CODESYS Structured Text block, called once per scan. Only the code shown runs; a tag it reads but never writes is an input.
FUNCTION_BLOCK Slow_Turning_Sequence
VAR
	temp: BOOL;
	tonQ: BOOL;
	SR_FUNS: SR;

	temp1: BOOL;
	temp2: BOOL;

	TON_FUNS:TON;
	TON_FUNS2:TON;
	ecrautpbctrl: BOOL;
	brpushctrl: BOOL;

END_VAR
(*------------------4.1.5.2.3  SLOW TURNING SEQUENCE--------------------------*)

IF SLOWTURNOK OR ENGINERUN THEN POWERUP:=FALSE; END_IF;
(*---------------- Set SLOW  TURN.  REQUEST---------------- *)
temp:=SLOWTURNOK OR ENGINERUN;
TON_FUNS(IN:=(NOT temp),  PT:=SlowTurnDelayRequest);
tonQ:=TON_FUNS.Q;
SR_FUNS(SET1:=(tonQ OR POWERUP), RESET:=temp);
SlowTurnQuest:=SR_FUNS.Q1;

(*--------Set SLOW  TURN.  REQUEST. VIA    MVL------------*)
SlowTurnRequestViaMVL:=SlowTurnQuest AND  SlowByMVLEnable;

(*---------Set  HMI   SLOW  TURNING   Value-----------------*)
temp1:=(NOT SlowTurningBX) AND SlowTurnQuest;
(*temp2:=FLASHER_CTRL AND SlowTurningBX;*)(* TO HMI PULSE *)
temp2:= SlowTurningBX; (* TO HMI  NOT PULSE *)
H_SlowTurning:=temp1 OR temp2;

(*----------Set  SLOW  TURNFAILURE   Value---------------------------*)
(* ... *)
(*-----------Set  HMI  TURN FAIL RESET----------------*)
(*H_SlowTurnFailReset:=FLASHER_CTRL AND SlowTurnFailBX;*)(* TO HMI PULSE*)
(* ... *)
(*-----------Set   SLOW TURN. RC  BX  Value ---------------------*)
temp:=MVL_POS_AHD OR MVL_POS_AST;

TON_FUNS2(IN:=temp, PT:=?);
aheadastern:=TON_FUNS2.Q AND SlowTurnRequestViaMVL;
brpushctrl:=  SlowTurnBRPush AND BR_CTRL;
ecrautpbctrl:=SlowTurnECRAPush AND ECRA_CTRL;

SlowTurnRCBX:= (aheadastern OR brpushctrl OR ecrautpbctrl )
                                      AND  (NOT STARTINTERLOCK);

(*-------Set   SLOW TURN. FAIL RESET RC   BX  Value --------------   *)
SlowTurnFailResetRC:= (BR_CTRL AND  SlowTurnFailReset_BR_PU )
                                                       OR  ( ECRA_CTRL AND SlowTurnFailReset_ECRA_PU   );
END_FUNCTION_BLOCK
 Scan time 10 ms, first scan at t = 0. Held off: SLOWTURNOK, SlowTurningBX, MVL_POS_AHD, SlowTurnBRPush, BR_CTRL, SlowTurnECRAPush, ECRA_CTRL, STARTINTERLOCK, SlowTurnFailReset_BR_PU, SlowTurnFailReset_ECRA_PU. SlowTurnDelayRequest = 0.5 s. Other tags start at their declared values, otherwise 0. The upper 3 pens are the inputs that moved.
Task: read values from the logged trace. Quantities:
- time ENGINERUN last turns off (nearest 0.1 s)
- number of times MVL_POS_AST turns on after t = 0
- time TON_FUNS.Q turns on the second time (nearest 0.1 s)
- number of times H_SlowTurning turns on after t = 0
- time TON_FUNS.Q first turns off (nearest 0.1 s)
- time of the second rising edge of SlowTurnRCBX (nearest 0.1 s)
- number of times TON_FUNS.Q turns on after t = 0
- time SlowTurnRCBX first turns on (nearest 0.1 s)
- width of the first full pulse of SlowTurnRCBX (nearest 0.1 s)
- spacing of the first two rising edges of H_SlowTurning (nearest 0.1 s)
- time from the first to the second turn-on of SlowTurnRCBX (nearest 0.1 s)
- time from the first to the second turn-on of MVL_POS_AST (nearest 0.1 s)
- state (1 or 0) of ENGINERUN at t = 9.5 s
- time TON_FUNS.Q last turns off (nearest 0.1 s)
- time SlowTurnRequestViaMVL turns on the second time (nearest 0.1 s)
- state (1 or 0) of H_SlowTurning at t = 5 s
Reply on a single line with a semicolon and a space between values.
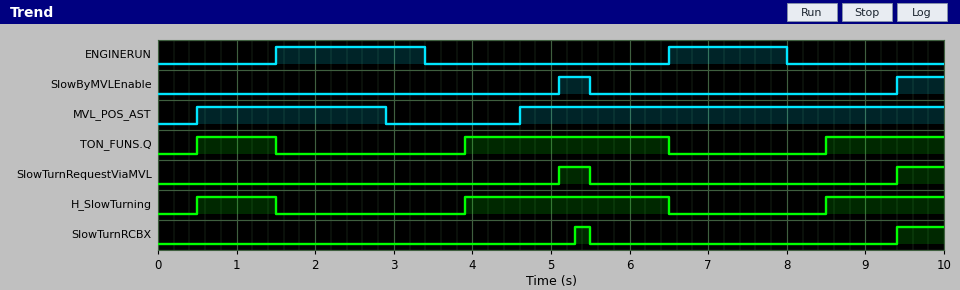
8.0 s; 2; 3.9 s; 3; 1.5 s; 9.4 s; 3; 5.3 s; 0.2 s; 3.4 s; 4.1 s; 4.1 s; 0; 6.5 s; 9.4 s; 1
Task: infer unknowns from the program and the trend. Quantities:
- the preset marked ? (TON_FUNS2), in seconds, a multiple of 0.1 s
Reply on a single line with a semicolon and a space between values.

0.7 s
